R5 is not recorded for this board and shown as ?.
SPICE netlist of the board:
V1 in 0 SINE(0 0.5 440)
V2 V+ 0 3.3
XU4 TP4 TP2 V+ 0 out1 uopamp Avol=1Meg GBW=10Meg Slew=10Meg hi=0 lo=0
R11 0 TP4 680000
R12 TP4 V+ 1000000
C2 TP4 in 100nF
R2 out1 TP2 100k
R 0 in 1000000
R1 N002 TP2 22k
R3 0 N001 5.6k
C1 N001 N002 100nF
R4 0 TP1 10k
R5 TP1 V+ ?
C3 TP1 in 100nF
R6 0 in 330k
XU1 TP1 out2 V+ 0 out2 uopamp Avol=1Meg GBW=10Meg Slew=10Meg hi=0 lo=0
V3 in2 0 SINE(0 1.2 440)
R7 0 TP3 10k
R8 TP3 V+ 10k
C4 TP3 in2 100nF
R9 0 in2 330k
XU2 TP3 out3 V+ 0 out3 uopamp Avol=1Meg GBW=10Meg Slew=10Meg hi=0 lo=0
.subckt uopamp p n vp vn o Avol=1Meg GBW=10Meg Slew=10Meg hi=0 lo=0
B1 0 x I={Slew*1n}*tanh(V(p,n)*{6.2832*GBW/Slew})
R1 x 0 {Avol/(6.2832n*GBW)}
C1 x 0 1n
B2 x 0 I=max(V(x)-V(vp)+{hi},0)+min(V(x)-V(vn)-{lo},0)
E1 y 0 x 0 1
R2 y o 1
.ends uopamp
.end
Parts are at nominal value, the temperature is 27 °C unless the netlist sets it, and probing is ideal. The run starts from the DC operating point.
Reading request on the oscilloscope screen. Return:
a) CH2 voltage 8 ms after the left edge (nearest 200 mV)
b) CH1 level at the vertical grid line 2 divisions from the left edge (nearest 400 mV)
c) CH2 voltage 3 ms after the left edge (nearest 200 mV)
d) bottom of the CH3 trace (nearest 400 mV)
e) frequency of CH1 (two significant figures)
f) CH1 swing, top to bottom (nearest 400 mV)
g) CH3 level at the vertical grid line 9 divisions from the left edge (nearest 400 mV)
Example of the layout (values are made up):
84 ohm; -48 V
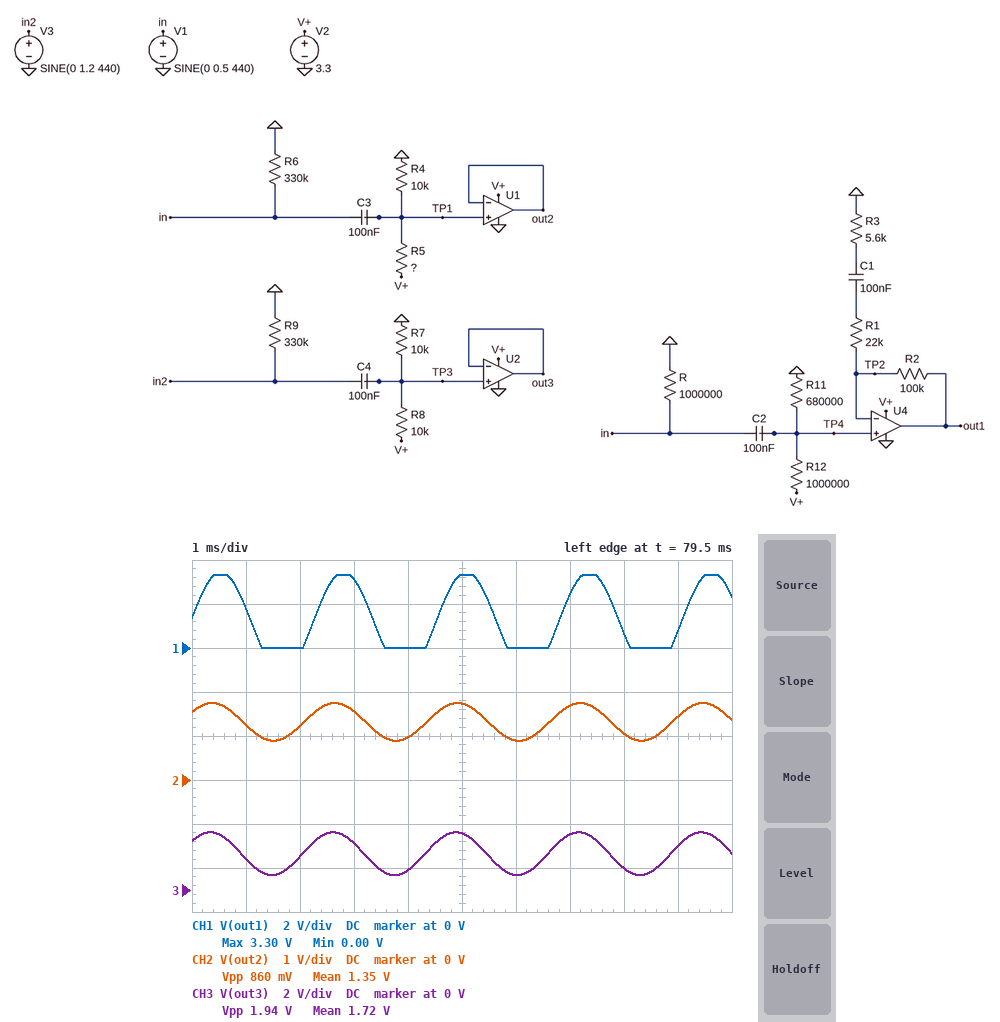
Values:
1.0 V; 0 V; 1.6 V; 800 mV; 440 Hz; 3.2 V; 2.0 V
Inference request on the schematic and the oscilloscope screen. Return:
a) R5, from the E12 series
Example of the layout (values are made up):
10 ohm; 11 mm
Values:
15 kΩ
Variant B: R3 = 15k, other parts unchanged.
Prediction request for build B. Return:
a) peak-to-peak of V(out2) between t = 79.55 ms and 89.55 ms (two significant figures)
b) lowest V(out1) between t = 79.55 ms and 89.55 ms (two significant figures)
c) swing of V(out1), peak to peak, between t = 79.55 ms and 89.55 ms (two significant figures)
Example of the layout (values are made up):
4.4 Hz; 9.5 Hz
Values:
860 mV; -7.5 mV; 3.1 V
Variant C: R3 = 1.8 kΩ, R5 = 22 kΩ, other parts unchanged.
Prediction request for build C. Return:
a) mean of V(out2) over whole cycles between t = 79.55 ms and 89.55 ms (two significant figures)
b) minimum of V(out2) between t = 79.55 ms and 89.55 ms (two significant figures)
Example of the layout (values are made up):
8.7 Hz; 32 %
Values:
1.0 V; 590 mV
